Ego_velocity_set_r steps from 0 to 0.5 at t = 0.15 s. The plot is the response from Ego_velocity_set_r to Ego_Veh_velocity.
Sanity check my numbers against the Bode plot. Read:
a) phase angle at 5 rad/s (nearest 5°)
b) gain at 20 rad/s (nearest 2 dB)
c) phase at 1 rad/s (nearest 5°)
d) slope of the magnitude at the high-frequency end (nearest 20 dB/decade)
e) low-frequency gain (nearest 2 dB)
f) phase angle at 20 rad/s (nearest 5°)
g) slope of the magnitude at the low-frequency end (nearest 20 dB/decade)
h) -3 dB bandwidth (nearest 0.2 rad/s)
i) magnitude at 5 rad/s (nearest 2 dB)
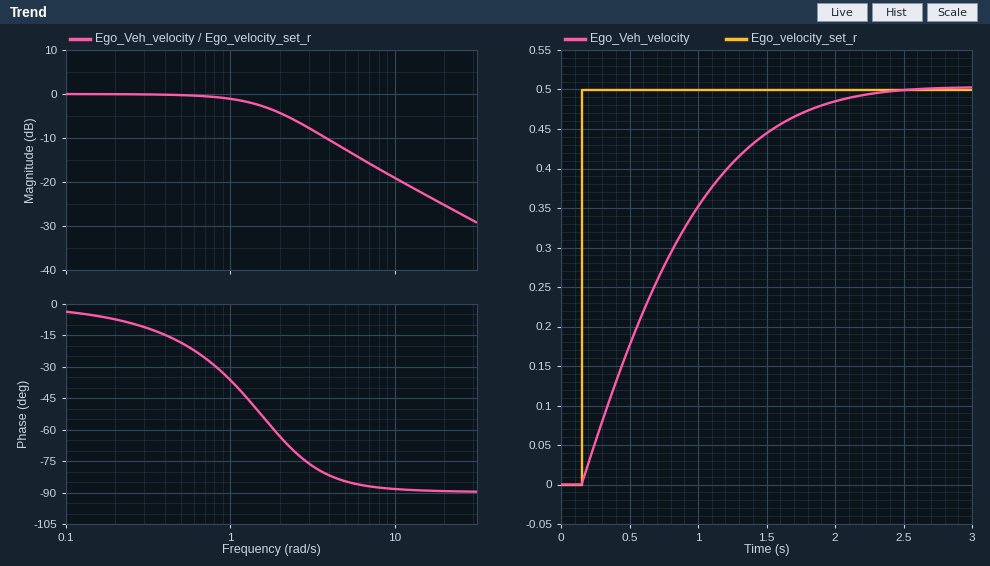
-85°
-26 dB
-35°
-20 dB/decade
0 dB
-90°
0 dB/decade
1.6 rad/s
-12 dB
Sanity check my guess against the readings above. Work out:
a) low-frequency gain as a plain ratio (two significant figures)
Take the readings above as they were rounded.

1.0
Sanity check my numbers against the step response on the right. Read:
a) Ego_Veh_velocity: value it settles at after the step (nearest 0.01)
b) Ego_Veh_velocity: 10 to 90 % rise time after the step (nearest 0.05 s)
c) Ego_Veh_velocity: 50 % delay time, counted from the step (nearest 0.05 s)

0.50
1.30 s
0.55 s
